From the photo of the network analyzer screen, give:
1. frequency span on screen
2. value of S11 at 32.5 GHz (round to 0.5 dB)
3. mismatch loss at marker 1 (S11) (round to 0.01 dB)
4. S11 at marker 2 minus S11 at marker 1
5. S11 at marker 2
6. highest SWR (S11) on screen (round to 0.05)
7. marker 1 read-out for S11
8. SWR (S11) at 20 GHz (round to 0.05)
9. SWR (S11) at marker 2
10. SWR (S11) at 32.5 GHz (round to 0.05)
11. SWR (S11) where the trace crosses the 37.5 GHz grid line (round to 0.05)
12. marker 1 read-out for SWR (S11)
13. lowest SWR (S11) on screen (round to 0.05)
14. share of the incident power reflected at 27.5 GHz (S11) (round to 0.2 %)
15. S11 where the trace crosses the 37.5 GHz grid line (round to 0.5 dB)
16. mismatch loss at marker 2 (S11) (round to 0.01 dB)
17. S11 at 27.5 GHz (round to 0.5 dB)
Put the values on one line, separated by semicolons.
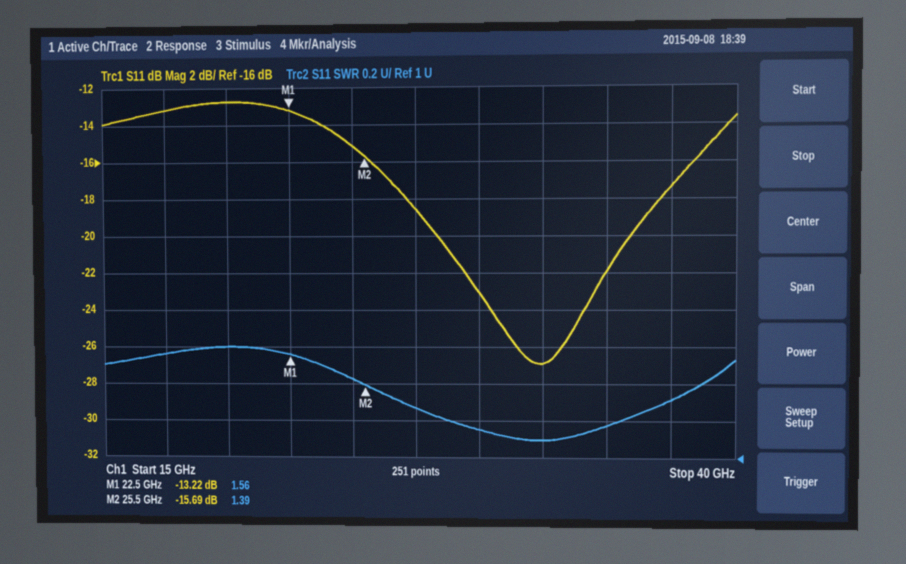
25 GHz; -27.0 dB; 0.21 dB; -2.47 dB; -15.69 dB; 1.60; -13.22 dB; 1.60; 1.39; 1.10; 1.30; 1.56; 1.10; 1.4 %; -17.5 dB; 0.12 dB; -18.5 dB
